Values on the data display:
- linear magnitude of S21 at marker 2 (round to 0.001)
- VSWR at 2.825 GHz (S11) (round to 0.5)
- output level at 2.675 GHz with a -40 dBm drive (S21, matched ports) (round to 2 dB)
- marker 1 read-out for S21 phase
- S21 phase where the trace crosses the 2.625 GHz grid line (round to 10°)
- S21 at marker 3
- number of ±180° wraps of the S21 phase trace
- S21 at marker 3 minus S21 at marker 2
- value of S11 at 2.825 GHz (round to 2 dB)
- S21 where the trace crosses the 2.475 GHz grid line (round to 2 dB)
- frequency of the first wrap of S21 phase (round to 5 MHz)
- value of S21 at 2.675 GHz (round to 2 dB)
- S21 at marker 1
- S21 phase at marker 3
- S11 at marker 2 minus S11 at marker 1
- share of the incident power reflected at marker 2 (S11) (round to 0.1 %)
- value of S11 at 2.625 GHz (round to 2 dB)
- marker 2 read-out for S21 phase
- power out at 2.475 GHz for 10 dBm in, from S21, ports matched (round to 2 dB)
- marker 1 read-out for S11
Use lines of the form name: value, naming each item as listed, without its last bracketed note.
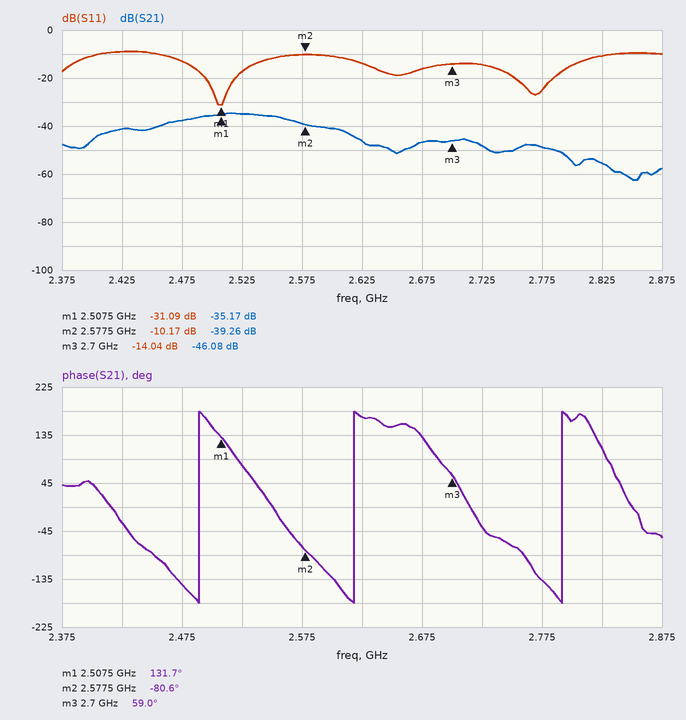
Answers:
linear magnitude of S21 at marker 2: 0.011
VSWR at 2.825 GHz (S11): 2.0
output level at 2.675 GHz with a -40 dBm drive (S21, matched ports): -86 dBm
marker 1 read-out for S21 phase: 131.7°
S21 phase where the trace crosses the 2.625 GHz grid line: 170°
S21 at marker 3: -46.08 dB
number of ±180° wraps of the S21 phase trace: 3
S21 at marker 3 minus S21 at marker 2: -6.82 dB
value of S11 at 2.825 GHz: -10 dB
S21 where the trace crosses the 2.475 GHz grid line: -38 dB
frequency of the first wrap of S21 phase: 2.490 GHz
value of S21 at 2.675 GHz: -46 dB
S21 at marker 1: -35.17 dB
S21 phase at marker 3: 59.0°
S11 at marker 2 minus S11 at marker 1: 20.92 dB
share of the incident power reflected at marker 2 (S11): 9.6 %
value of S11 at 2.625 GHz: -14 dB
marker 2 read-out for S21 phase: -80.6°
power out at 2.475 GHz for 10 dBm in, from S21, ports matched: -28 dBm
marker 1 read-out for S11: -31.09 dB
